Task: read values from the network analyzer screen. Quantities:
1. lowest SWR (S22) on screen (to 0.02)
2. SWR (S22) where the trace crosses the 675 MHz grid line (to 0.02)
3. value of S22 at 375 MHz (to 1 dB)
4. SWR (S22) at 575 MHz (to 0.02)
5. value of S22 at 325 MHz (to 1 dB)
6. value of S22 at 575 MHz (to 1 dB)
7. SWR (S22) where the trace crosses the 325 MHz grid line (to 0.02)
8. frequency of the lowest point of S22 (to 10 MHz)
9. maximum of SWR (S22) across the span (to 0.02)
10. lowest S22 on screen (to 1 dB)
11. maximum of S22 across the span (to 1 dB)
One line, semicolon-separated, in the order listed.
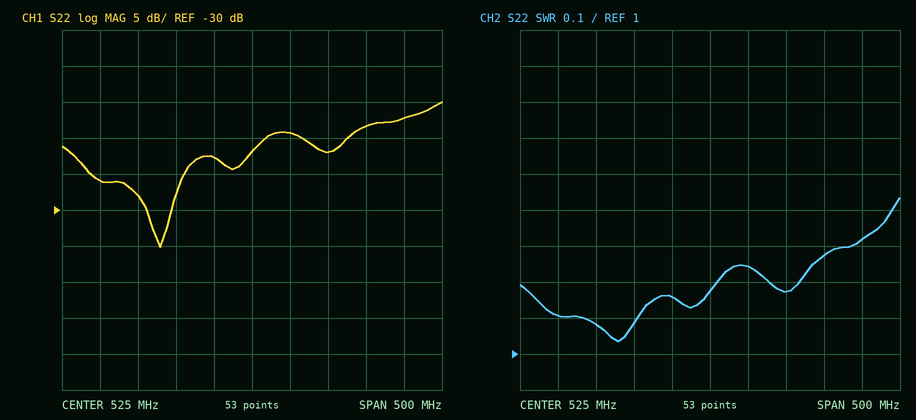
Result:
1.04; 1.28; -28 dB; 1.24; -26 dB; -19 dB; 1.10; 400 MHz; 1.44; -35 dB; -15 dB
